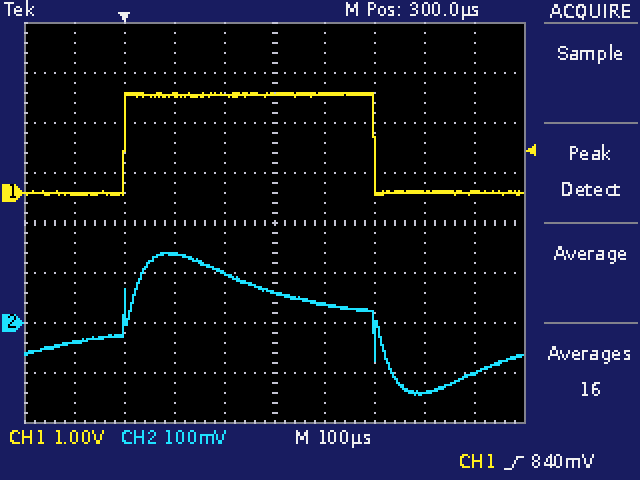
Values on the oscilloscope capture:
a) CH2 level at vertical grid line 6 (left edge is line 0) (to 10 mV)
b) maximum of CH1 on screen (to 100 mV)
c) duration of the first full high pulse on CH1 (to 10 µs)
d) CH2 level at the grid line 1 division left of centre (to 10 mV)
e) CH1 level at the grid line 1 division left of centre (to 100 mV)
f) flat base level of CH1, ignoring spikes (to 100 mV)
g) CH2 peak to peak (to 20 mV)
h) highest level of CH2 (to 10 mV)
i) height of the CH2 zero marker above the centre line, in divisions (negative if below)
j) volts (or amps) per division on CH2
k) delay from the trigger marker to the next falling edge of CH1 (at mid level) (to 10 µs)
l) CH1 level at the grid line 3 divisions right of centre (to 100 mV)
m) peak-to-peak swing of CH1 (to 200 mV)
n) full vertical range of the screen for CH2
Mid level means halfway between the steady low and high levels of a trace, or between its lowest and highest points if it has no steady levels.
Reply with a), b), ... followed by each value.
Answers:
a) 40 mV
b) 2.0 V
c) 500 µs
d) 100 mV
e) 2.0 V
f) 0.0 V
g) 280 mV
h) 140 mV
i) -2.0 div
j) 100 mV
k) 500 µs
l) 0.0 V
m) 2.0 V
n) 800 mV
